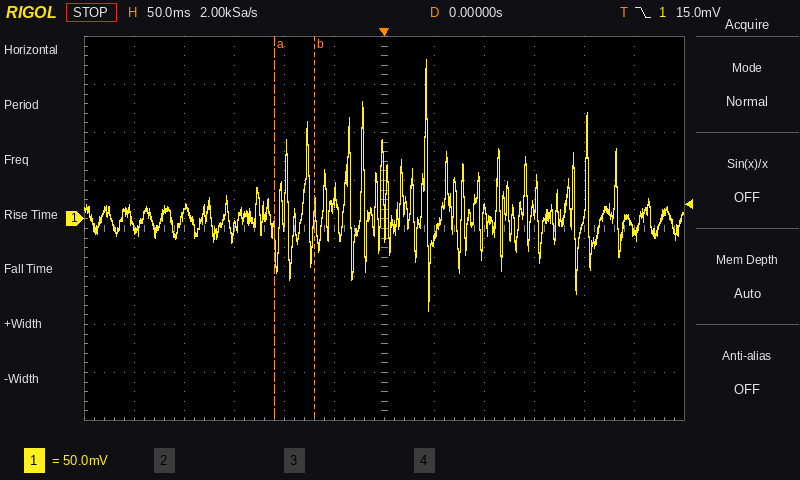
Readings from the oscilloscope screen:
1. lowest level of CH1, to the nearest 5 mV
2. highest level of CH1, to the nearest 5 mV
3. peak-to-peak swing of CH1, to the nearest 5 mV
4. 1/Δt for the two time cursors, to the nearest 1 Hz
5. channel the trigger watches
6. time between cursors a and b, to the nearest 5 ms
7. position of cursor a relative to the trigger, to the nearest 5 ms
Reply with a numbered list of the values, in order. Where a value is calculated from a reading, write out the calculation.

1. -95 mV
2. 165 mV
3. 165 mV − (-95 mV) = 260 mV
4. 1 / 40 ms ≈ 25 Hz
5. CH1
6. 40 ms
7. -110 ms
